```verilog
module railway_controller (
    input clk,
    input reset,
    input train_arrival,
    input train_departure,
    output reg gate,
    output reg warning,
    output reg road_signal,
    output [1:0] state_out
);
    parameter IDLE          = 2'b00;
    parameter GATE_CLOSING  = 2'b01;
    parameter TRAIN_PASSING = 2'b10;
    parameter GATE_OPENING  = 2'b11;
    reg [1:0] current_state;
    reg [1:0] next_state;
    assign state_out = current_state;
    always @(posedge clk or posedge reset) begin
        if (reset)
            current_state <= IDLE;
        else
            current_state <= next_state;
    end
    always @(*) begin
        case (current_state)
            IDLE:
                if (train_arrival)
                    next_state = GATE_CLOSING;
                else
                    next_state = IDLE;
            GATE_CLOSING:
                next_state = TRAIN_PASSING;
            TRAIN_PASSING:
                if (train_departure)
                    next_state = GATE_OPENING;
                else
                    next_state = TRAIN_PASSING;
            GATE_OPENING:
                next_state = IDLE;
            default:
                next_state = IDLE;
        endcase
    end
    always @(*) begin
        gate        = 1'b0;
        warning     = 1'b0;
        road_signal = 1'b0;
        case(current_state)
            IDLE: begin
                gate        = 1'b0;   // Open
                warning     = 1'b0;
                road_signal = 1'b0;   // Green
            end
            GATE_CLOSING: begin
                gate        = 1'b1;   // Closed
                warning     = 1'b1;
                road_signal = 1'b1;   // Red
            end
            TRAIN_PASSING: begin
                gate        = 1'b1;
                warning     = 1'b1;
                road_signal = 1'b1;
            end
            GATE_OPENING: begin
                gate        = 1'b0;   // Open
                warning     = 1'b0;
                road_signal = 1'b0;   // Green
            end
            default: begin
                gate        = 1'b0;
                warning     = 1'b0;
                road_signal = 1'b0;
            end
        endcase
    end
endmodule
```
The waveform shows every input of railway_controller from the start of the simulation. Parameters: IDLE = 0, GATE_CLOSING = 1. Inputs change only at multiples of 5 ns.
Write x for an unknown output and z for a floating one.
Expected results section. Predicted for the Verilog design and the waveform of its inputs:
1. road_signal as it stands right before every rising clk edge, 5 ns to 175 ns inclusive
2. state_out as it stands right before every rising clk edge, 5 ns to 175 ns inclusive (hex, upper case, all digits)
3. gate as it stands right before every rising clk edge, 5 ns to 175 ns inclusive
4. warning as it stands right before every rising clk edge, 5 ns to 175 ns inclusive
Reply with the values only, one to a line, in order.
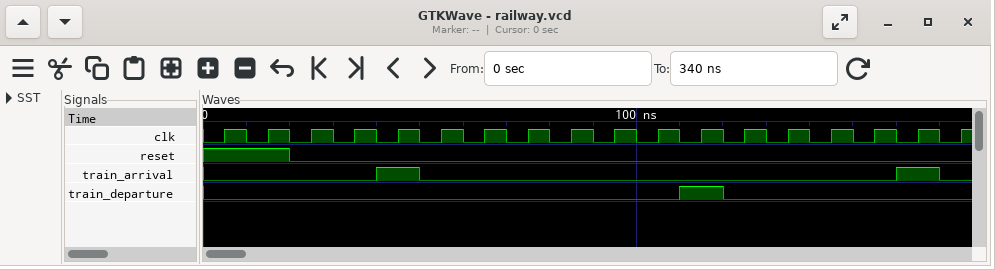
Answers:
0 0 0 0 0 1 1 1 1 1 1 1 0 0 0 0 0 1
0, 0, 0, 0, 0, 1, 2, 2, 2, 2, 2, 2, 3, 0, 0, 0, 0, 1
0 0 0 0 0 1 1 1 1 1 1 1 0 0 0 0 0 1
0 0 0 0 0 1 1 1 1 1 1 1 0 0 0 0 0 1
